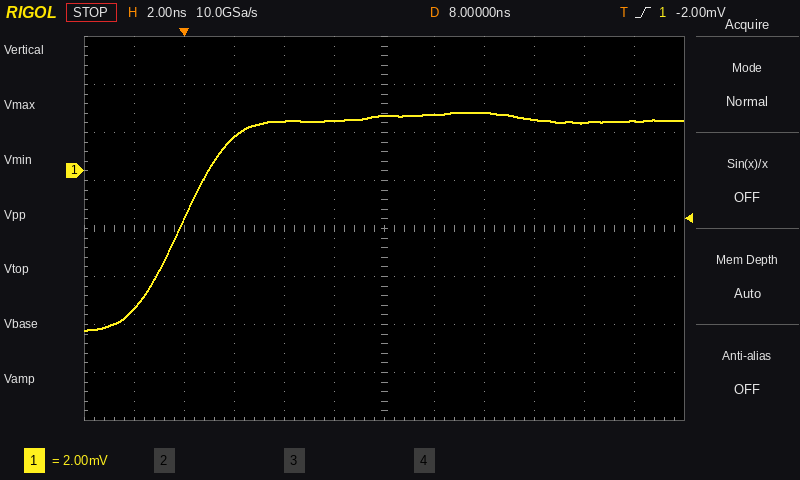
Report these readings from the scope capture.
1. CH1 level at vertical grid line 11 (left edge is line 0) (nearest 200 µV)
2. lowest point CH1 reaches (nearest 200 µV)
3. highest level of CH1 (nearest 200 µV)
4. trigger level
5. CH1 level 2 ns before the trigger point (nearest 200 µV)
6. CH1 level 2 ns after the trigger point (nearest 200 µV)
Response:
2.0 mV
-6.6 mV
2.4 mV
-2.00 mV
-5.8 mV
1.4 mV
